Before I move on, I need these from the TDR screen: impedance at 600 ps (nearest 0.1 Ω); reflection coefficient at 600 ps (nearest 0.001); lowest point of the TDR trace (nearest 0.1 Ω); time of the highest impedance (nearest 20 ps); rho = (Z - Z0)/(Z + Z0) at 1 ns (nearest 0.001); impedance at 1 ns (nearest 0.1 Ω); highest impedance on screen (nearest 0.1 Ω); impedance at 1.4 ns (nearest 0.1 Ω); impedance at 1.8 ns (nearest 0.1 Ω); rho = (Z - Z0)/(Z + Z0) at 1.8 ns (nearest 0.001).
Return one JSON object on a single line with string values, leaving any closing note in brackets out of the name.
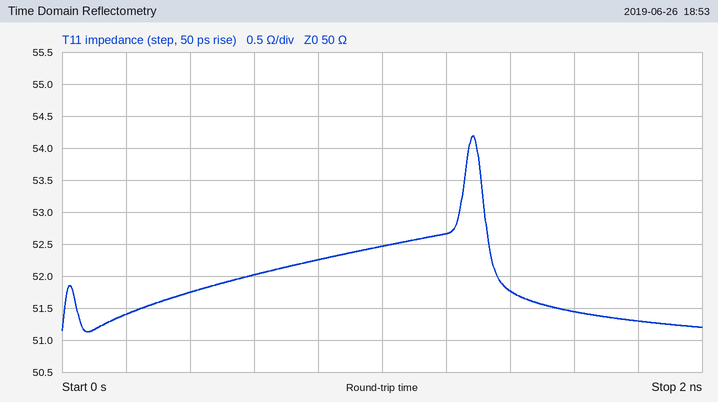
{"impedance at 600 ps": "52.0 Ω", "reflection coefficient at 600 ps": "+0.020", "lowest point of the TDR trace": "51.1 Ω", "time of the highest impedance": "1.28 ns", "rho = (Z - Z0)/(Z + Z0) at 1 ns": "+0.024", "impedance at 1 ns": "52.5 Ω", "highest impedance on screen": "54.2 Ω", "impedance at 1.4 ns": "51.8 Ω", "impedance at 1.8 ns": "51.3 Ω", "rho = (Z - Z0)/(Z + Z0) at 1.8 ns": "+0.013"}
